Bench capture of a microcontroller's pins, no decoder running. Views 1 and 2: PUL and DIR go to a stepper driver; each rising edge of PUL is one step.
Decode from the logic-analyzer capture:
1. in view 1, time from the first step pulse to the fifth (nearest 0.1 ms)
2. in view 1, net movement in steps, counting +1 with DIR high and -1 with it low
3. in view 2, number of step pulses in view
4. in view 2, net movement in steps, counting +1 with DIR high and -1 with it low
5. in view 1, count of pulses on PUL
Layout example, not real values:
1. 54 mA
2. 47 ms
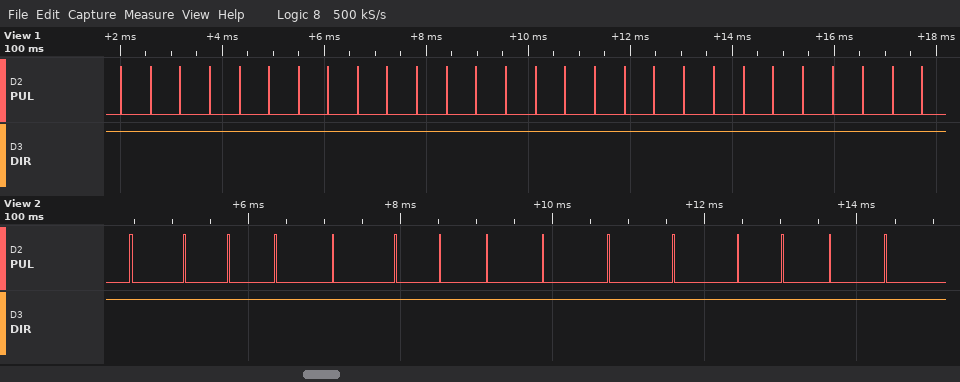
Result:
1. 2.3 ms
2. +28
3. 15
4. +15
5. 28
